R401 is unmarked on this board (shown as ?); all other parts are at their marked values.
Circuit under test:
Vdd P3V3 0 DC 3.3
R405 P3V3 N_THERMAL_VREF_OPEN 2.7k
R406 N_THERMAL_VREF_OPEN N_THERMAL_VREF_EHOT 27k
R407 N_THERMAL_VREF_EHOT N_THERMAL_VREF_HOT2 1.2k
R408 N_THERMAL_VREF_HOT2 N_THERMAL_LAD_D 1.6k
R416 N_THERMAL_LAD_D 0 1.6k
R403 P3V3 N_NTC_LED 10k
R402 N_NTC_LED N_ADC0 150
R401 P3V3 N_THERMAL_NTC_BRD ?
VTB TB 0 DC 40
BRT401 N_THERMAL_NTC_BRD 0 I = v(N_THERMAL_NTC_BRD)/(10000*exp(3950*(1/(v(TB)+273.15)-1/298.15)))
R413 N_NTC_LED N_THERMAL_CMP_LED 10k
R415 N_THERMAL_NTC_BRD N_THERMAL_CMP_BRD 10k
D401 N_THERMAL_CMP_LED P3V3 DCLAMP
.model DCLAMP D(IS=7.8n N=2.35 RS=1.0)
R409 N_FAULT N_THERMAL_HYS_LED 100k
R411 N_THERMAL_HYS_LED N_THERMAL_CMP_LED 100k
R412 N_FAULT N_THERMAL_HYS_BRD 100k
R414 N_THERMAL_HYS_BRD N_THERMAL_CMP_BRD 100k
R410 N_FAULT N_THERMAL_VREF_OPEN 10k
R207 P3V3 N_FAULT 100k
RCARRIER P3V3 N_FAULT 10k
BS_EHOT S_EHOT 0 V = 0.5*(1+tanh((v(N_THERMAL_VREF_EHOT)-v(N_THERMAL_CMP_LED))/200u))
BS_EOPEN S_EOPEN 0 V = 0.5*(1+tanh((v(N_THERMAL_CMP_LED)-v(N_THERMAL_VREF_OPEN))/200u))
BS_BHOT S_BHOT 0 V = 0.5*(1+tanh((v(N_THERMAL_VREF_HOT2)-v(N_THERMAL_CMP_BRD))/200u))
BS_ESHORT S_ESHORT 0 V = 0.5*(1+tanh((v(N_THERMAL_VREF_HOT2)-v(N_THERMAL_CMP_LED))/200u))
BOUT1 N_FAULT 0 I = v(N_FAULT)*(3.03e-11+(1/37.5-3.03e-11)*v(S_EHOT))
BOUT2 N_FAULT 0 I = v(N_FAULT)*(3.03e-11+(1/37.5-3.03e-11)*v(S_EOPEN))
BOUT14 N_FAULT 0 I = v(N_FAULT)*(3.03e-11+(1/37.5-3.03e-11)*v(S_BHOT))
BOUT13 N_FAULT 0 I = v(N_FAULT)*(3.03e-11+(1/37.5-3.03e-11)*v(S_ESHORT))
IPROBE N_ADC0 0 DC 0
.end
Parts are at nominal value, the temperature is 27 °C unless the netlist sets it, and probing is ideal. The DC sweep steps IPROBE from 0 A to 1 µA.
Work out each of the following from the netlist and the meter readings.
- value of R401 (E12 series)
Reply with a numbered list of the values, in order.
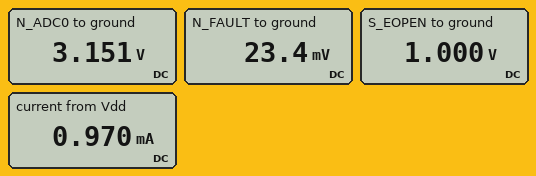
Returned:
1. 6.8 kΩ
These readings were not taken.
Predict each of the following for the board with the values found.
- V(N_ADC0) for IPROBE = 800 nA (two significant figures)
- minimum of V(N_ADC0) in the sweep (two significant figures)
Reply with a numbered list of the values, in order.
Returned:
1. 3.1 V
2. 3.1 V
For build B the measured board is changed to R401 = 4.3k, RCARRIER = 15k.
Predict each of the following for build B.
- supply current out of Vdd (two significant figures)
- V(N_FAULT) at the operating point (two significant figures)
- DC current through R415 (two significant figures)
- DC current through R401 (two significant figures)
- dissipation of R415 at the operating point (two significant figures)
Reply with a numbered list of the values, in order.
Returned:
1. 930 µA
2. 19 mV
3. 8.5 µA
4. 350 µA
5. 720 nW
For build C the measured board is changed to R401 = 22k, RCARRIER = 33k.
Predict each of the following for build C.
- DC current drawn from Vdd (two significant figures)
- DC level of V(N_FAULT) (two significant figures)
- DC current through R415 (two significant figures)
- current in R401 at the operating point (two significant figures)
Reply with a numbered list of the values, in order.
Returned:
1. 590 µA
2. 15 mV
3. 2.9 µA
4. 120 µA
